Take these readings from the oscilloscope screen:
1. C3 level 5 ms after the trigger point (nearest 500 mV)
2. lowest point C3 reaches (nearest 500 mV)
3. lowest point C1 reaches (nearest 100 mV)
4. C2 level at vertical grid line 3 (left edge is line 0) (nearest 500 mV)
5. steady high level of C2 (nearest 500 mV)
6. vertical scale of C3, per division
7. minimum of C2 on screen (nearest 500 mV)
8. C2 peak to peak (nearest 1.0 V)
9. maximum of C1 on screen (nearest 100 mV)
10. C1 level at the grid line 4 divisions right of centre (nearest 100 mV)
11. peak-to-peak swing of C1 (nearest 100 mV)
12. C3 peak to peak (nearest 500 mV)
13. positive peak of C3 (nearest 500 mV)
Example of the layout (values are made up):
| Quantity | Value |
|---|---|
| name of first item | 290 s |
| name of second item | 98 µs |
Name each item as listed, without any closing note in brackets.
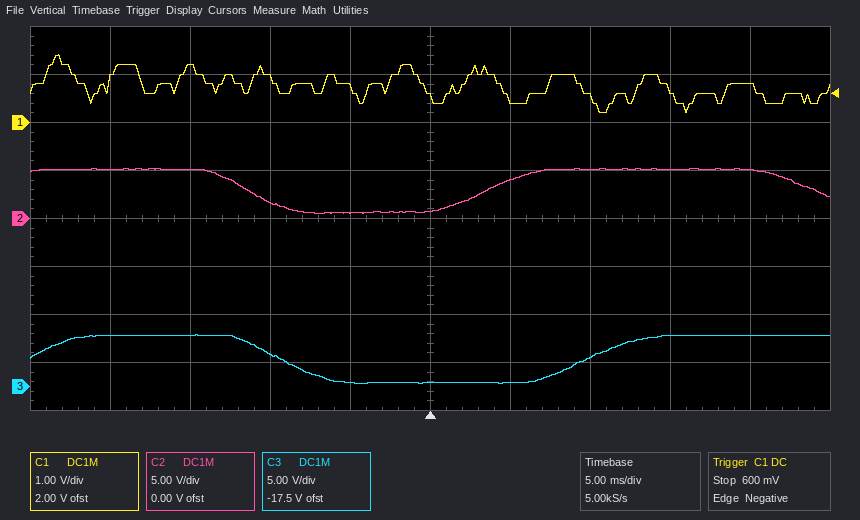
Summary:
| Quantity | Value |
|---|---|
| C3 level 5 ms after the trigger point | 500 mV |
| lowest point C3 reaches | 500 mV |
| lowest point C1 reaches | 200 mV |
| C2 level at vertical grid line 3 (left edge is line 0) | 1.5 V |
| steady high level of C2 | 5.0 V |
| vertical scale of C3, per division | 5 V |
| minimum of C2 on screen | 500 mV |
| C2 peak to peak | 5.0 V |
| maximum of C1 on screen | 1.4 V |
| C1 level at the grid line 4 divisions right of centre | 800 mV |
| peak-to-peak swing of C1 | 1.2 V |
| C3 peak to peak | 5.0 V |
| positive peak of C3 | 5.5 V |
